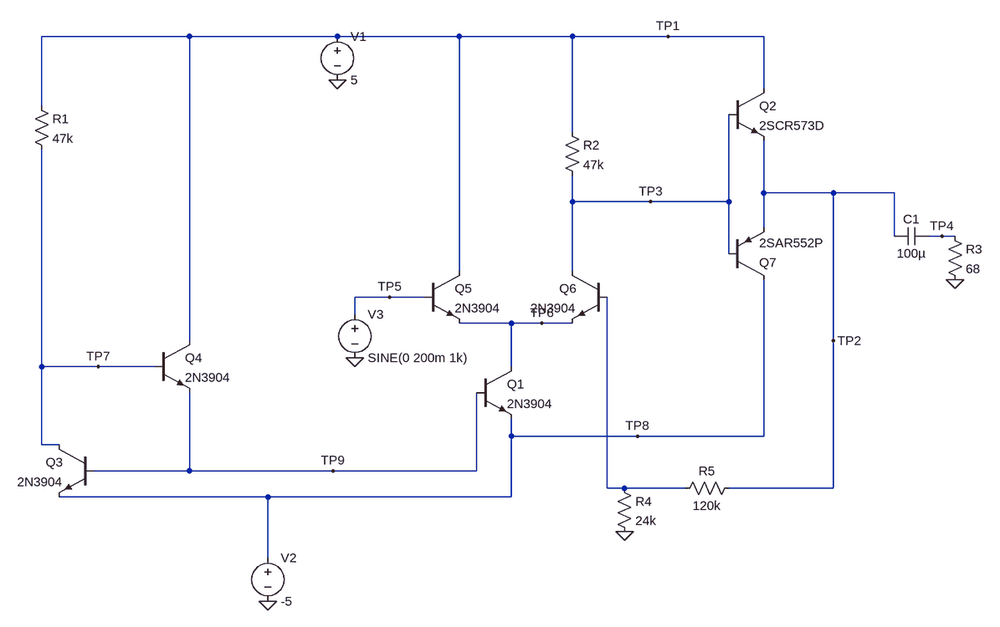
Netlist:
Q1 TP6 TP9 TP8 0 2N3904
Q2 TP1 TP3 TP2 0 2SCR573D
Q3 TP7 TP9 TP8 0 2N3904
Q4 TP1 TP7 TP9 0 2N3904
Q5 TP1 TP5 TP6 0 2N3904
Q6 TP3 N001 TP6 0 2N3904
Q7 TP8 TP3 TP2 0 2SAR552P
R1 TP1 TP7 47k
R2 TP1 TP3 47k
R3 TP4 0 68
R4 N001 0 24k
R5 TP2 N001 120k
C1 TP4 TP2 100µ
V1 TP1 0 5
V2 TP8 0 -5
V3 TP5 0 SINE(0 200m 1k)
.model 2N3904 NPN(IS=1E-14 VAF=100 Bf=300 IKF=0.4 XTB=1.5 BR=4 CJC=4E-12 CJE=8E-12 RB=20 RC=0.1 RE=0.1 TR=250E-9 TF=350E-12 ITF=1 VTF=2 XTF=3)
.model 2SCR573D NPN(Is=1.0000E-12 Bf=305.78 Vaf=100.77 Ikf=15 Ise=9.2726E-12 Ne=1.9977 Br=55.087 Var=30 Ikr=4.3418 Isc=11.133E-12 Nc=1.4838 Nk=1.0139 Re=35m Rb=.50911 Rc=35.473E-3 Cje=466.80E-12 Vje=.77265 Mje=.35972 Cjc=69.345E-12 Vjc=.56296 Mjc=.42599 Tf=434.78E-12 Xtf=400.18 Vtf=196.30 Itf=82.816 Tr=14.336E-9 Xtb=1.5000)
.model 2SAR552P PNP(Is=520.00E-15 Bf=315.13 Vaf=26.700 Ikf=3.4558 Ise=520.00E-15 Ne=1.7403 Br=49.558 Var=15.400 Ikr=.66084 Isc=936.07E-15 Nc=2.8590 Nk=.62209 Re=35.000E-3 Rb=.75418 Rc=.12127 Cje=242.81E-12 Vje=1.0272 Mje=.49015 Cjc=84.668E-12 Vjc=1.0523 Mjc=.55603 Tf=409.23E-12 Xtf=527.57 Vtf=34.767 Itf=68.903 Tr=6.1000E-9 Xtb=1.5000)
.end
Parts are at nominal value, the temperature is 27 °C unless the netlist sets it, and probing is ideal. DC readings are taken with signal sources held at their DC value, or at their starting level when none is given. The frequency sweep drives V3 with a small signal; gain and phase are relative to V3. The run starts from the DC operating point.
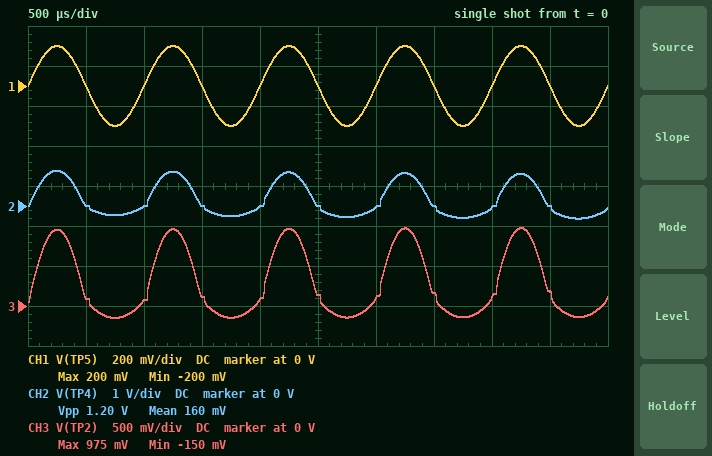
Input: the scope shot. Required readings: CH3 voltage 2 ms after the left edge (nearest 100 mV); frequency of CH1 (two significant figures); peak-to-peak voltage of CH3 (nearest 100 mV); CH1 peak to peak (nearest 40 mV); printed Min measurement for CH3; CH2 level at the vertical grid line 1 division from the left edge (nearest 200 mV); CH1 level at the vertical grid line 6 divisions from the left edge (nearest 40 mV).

100 mV
1.0 kHz
1.1 V
400 mV
-150 mV
0 V
0 V
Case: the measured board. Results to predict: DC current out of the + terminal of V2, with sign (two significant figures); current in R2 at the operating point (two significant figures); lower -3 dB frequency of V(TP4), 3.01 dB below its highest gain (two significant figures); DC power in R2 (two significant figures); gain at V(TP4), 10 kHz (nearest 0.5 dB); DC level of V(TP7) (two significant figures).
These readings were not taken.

-390 µA
98 µA
520 mHz
450 µW
-21.0 dB
-3.9 V
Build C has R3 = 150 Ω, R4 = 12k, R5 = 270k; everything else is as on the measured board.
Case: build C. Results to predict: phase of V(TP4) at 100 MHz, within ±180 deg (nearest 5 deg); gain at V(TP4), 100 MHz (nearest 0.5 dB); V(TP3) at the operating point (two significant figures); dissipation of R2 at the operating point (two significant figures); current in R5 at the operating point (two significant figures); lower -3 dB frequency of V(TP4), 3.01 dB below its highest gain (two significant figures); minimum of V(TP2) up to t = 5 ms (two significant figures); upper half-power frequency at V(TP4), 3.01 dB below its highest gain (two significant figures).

-15 deg
-29.0 dB
440 mV
440 µW
390 nA
200 mHz
-170 mV
1.7 MHz
